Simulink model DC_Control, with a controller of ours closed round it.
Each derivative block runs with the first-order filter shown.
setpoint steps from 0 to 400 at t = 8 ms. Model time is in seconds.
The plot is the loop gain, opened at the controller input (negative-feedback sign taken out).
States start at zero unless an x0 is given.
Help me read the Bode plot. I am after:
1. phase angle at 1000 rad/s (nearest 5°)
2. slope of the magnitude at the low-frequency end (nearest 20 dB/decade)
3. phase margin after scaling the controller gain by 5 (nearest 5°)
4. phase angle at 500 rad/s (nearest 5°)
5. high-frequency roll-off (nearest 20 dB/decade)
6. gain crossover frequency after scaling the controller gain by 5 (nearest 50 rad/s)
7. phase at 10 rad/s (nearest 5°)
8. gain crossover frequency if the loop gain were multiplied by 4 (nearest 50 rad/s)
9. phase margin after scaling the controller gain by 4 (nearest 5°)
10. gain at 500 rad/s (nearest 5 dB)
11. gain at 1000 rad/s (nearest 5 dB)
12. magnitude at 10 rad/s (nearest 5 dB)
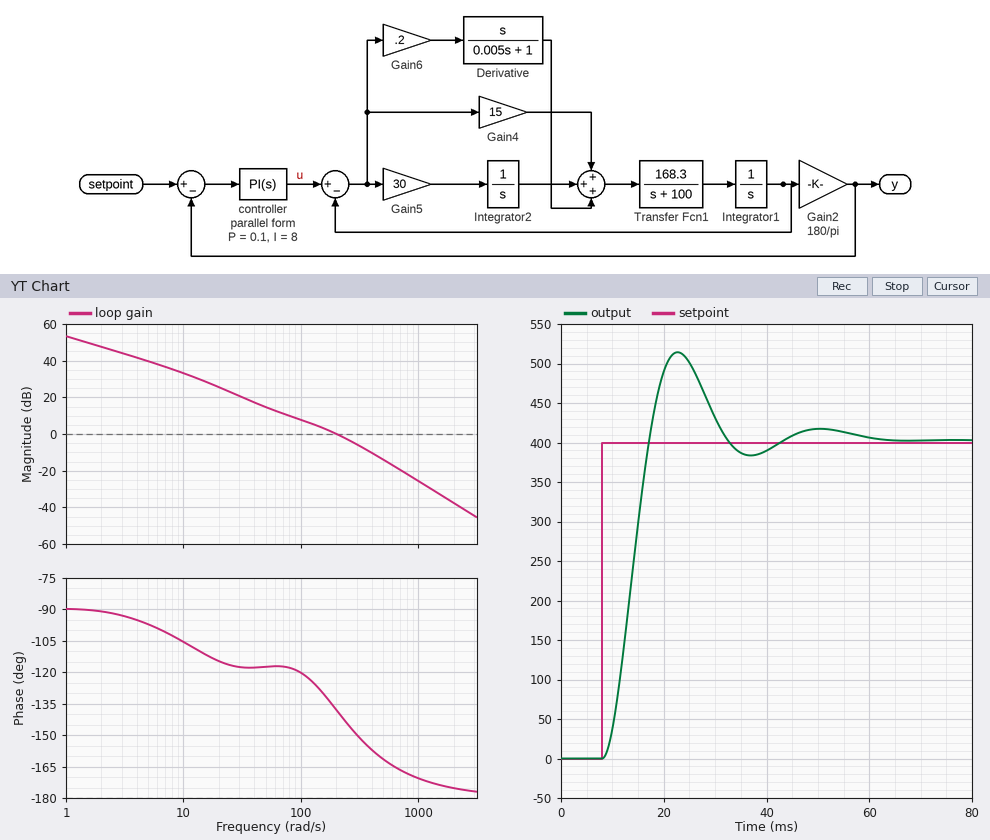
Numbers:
-170°
-20 dB/decade
20°
-160°
-40 dB/decade
500 rad/s
-105°
450 rad/s
20°
-15 dB
-25 dB
35 dB
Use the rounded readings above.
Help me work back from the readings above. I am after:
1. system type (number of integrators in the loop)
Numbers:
1
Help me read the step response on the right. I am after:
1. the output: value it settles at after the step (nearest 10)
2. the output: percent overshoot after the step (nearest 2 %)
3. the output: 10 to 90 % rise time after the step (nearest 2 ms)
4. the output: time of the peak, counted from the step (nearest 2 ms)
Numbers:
400
28 %
6 ms
14 ms
